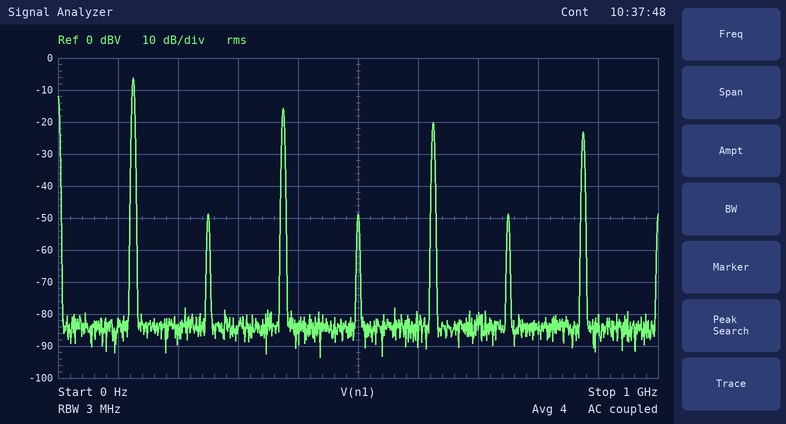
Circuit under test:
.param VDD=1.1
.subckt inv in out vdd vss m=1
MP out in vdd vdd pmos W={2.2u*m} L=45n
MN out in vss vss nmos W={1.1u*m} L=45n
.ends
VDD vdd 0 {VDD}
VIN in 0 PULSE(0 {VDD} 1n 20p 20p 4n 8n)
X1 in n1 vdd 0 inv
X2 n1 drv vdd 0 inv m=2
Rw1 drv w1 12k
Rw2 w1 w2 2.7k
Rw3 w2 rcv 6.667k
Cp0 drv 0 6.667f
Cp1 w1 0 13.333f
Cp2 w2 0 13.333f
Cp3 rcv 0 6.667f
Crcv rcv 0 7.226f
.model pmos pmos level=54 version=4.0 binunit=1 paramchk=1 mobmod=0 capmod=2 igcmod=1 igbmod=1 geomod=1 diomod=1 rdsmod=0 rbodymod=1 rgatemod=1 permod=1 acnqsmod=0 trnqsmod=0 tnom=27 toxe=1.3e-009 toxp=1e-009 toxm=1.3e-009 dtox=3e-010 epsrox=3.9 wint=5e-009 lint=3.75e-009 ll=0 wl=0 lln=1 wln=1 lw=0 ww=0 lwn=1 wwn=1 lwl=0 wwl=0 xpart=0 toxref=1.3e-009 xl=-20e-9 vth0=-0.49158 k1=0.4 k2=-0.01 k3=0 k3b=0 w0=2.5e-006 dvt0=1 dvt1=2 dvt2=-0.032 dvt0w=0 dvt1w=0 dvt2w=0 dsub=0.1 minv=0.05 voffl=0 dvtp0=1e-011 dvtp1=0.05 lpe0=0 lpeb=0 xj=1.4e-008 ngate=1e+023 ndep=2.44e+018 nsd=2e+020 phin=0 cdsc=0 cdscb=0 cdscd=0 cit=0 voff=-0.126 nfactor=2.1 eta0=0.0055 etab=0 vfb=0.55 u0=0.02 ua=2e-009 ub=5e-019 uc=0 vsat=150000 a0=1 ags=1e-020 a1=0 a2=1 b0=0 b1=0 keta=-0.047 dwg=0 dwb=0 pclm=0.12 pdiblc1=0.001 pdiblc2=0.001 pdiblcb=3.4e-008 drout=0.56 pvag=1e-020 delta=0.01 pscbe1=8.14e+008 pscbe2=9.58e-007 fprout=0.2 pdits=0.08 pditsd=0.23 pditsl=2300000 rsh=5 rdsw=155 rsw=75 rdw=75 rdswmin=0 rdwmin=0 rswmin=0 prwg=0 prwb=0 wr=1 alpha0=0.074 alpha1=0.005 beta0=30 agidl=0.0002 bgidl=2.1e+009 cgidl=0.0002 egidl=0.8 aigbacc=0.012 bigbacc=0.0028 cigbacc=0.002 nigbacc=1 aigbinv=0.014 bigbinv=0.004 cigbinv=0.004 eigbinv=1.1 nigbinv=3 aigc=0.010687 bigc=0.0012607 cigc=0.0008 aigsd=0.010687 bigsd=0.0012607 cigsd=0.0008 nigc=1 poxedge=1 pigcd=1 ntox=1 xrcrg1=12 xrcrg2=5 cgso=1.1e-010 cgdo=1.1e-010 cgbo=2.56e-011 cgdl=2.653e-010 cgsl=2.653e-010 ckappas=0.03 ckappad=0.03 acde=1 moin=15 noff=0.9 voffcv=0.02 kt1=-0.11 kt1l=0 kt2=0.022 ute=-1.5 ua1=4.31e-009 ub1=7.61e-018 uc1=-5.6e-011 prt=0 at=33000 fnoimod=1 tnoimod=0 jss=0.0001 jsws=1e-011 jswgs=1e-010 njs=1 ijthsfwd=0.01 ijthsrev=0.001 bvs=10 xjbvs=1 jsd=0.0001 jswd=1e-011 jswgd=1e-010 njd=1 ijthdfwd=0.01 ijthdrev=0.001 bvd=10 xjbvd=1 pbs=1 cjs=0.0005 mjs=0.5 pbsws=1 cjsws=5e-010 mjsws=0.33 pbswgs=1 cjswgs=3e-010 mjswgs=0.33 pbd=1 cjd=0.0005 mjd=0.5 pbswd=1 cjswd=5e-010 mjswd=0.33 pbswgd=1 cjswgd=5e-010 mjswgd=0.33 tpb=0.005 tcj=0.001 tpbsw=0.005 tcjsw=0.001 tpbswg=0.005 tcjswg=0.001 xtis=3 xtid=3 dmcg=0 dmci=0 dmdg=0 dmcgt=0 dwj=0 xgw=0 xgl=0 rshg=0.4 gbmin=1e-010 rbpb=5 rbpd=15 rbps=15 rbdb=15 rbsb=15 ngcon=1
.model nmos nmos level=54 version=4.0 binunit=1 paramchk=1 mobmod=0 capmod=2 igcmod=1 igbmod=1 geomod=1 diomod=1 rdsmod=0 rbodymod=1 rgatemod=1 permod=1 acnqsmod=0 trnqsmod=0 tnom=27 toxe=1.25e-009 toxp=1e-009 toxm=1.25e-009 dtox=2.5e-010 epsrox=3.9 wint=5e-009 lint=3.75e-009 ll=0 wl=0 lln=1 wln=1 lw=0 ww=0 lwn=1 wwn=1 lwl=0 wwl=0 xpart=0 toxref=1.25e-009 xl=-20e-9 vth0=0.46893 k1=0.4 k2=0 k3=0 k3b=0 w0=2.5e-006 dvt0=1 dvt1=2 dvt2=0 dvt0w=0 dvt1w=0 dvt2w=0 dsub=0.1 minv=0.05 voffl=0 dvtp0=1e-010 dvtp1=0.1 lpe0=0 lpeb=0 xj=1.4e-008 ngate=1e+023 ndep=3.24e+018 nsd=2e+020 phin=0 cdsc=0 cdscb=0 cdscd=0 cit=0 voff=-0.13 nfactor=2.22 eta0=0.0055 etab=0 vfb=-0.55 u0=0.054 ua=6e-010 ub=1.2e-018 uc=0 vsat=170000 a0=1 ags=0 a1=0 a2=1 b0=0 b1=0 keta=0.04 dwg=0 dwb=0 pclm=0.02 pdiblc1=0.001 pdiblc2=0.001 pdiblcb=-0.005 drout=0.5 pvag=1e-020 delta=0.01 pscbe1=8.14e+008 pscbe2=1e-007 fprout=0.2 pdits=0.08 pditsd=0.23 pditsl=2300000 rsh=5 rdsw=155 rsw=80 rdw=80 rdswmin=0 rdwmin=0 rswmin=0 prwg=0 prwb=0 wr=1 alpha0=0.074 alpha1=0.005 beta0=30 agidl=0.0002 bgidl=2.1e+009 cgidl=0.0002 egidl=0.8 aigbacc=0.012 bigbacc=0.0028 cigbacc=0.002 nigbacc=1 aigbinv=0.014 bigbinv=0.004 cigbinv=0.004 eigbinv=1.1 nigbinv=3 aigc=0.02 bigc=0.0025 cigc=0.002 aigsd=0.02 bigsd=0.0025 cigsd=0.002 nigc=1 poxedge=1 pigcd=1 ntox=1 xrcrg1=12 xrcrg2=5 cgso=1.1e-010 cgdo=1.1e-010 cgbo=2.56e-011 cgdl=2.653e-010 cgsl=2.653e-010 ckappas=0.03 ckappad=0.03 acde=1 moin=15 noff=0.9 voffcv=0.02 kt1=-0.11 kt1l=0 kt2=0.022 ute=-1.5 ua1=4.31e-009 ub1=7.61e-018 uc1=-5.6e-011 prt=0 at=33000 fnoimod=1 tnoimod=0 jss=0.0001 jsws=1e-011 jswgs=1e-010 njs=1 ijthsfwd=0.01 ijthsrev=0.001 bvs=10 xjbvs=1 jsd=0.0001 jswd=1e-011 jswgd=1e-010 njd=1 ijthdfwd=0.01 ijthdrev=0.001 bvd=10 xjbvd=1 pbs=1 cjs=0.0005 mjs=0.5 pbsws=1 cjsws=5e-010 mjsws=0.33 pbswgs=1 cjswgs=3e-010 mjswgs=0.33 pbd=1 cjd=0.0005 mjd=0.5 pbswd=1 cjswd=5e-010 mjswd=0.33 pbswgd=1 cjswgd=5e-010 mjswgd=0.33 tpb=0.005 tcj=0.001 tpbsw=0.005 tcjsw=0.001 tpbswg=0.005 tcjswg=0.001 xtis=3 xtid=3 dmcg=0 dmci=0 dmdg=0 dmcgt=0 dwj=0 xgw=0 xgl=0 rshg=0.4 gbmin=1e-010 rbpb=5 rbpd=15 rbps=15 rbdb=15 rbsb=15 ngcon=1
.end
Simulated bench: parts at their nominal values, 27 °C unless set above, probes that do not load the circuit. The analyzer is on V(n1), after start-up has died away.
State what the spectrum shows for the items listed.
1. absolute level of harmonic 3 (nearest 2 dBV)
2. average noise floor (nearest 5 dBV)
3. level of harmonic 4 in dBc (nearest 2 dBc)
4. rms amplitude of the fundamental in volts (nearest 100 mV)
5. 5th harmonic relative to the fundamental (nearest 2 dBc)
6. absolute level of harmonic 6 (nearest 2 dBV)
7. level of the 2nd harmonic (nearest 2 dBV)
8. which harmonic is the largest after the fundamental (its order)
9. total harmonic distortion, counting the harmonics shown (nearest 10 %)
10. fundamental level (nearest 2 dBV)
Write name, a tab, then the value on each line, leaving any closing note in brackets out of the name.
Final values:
absolute level of harmonic 3	-16 dBV
average noise floor	-85 dBV
level of harmonic 4 in dBc	-42 dBc
rms amplitude of the fundamental in volts	500 mV
5th harmonic relative to the fundamental	-14 dBc
absolute level of harmonic 6	-48 dBV
level of the 2nd harmonic	-48 dBV
which harmonic is the largest after the fundamental	3
total harmonic distortion, counting the harmonics shown	40 %
fundamental level	-6 dBV
